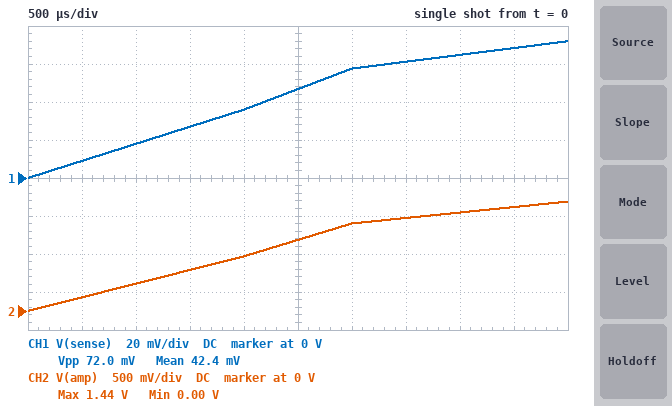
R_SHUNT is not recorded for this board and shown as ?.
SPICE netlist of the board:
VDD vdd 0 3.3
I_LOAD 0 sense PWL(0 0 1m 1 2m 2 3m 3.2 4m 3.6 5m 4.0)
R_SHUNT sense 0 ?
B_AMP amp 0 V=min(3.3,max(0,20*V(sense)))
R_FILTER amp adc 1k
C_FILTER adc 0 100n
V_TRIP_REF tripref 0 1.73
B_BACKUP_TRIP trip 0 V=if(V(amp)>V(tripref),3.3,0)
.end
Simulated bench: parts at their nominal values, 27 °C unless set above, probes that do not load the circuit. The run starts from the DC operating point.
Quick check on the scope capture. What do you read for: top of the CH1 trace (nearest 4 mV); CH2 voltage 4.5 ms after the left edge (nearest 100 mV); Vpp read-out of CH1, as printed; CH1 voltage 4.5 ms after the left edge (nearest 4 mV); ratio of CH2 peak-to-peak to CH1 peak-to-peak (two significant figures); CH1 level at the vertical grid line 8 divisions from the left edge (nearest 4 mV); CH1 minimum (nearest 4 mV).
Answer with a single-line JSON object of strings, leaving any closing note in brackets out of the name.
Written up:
{"top of the CH1 trace": "72 mV", "CH2 voltage 4.5 ms after the left edge": "1.4 V", "Vpp read-out of CH1, as printed": "72.0 mV", "CH1 voltage 4.5 ms after the left edge": "68 mV", "ratio of CH2 peak-to-peak to CH1 peak-to-peak": "20", "CH1 level at the vertical grid line 8 divisions from the left edge": "64 mV", "CH1 minimum": "0 V"}
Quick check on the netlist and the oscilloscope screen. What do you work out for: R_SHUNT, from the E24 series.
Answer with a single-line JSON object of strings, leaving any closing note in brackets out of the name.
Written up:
{"R_SHUNT, from the E24 series": "0.018 Ω"}
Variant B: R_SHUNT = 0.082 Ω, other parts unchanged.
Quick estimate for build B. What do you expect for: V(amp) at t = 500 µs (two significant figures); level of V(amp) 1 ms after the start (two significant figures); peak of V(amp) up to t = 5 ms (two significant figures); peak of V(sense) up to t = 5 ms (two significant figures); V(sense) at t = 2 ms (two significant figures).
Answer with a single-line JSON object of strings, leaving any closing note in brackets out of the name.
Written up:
{"V(amp) at t = 500 µs": "820 mV", "level of V(amp) 1 ms after the start": "1.6 V", "peak of V(amp) up to t = 5 ms": "3.3 V", "peak of V(sense) up to t = 5 ms": "330 mV", "V(sense) at t = 2 ms": "160 mV"}
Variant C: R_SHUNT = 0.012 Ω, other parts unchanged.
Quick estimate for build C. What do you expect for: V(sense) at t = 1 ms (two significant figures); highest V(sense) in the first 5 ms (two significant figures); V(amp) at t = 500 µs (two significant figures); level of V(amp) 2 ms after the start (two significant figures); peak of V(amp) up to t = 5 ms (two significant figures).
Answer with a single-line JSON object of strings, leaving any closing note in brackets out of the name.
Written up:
{"V(sense) at t = 1 ms": "12 mV", "highest V(sense) in the first 5 ms": "48 mV", "V(amp) at t = 500 µs": "120 mV", "level of V(amp) 2 ms after the start": "480 mV", "peak of V(amp) up to t = 5 ms": "960 mV"}
